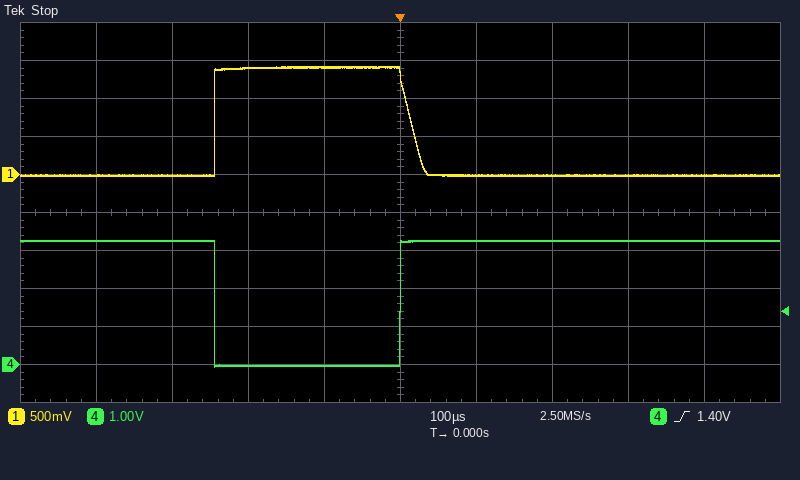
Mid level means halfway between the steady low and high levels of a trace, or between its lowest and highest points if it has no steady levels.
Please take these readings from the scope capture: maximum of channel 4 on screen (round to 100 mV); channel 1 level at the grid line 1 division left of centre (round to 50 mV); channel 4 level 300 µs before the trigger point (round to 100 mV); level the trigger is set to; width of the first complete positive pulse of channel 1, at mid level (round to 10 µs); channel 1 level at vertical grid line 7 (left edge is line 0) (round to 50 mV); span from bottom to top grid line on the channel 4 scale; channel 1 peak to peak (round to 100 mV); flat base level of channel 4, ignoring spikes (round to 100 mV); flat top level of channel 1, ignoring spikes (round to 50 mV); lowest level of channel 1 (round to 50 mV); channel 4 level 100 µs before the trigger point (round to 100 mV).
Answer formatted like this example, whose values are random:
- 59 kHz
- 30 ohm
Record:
- 3.3 V
- 1.40 V
- 3.3 V
- 1.40 V
- 260 µs
- 0 mV
- 10 V
- 1.40 V
- 0.0 V
- 1.40 V
- 0 mV
- 0.0 V
